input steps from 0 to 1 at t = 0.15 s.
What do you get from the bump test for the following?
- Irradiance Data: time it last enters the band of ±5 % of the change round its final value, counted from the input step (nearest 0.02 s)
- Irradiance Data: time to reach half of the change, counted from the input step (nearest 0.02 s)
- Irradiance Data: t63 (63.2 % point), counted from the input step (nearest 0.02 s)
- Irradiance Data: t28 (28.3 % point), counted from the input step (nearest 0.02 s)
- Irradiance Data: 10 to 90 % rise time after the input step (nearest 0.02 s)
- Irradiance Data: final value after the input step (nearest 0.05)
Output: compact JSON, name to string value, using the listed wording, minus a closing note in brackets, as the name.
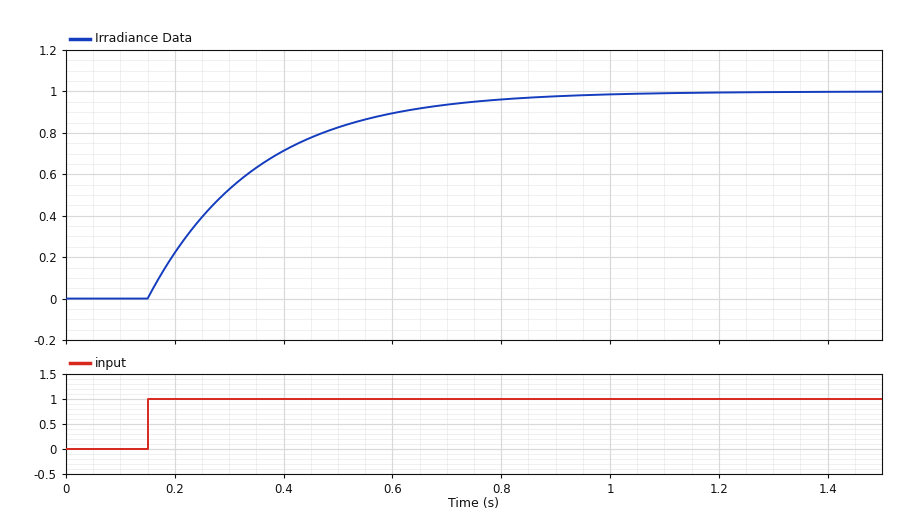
{"Irradiance Data: time it last enters the band of ±5 % of the change round its final value, counted from the input step": "0.60 s", "Irradiance Data: time to reach half of the change, counted from the input step": "0.14 s", "Irradiance Data: t63 (63.2 % point), counted from the input step": "0.20 s", "Irradiance Data: t28 (28.3 % point), counted from the input step": "0.06 s", "Irradiance Data: 10 to 90 % rise time after the input step": "0.44 s", "Irradiance Data: final value after the input step": "1.00"}
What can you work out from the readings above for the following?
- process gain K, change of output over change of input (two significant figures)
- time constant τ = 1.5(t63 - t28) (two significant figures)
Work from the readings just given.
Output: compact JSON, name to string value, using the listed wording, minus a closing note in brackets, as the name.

{"process gain K, change of output over change of input": "1.0", "time constant τ = 1.5(t63 - t28)": "0.21 s"}
